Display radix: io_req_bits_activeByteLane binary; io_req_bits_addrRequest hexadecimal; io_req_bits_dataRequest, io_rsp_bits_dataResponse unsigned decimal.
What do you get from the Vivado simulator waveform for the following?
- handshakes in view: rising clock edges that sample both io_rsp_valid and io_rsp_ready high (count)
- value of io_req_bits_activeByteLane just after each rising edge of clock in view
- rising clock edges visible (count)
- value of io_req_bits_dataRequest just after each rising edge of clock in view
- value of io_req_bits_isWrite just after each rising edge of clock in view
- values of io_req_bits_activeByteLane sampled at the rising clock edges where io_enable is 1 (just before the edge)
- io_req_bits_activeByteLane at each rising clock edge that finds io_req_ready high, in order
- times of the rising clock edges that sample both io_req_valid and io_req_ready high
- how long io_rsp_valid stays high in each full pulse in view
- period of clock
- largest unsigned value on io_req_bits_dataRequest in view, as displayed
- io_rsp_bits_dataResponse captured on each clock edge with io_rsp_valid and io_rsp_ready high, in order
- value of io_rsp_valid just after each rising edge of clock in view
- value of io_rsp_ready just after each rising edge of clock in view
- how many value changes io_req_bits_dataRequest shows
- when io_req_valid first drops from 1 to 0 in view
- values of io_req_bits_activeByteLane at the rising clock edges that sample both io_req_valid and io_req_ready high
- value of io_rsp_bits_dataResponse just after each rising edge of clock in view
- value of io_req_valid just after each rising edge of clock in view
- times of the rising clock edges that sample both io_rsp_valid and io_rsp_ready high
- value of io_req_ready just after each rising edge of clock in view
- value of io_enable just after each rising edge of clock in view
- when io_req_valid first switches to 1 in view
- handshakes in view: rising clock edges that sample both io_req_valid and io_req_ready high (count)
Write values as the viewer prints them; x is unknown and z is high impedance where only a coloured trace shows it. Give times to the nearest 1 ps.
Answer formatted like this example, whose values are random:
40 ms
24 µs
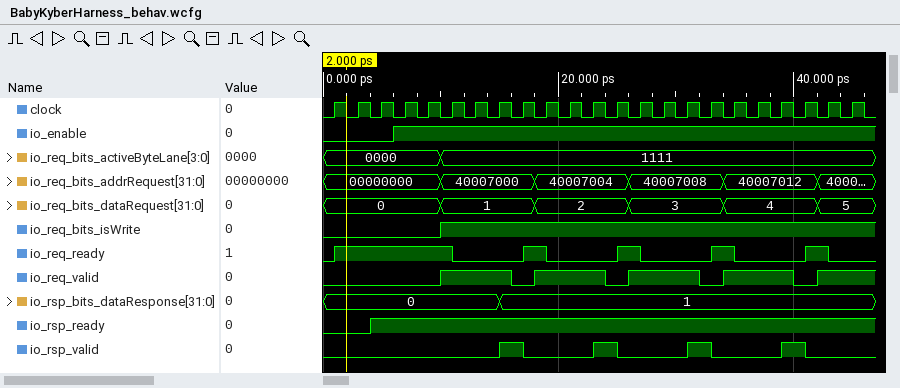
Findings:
4
0000, 0000, 0000, 0000, 0000, 1111, 1111, 1111, 1111, 1111, 1111, 1111, 1111, 1111, 1111, 1111, 1111, 1111, 1111, 1111, 1111, 1111, 1111
23
0, 0, 0, 0, 0, 1, 1, 1, 1, 2, 2, 2, 2, 3, 3, 3, 3, 4, 4, 4, 4, 5, 5
0 0 0 0 0 1 1 1 1 1 1 1 1 1 1 1 1 1 1 1 1 1 1
0000, 0000, 1111, 1111, 1111, 1111, 1111, 1111, 1111, 1111, 1111, 1111, 1111, 1111, 1111, 1111, 1111, 1111, 1111, 1111
0000, 0000, 0000, 0000, 1111, 1111, 1111, 1111, 1111
11 ps, 19 ps, 27 ps, 35 ps, 43 ps
2 ps, 2 ps, 2 ps, 2 ps
2 ps
5
1, 1, 1, 1
0 0 0 0 0 0 0 1 0 0 0 1 0 0 0 1 0 0 0 1 0 0 0
0 0 1 1 1 1 1 1 1 1 1 1 1 1 1 1 1 1 1 1 1 1 1
5
16 ps
1111, 1111, 1111, 1111, 1111
0, 0, 0, 0, 0, 0, 0, 1, 1, 1, 1, 1, 1, 1, 1, 1, 1, 1, 1, 1, 1, 1, 1
0 0 0 0 0 1 1 1 0 1 1 1 0 1 1 1 0 1 1 1 0 1 1
17 ps, 25 ps, 33 ps, 41 ps
1 1 1 1 1 0 0 0 1 0 0 0 1 0 0 0 1 0 0 0 1 0 0
0 0 0 1 1 1 1 1 1 1 1 1 1 1 1 1 1 1 1 1 1 1 1
10 ps
5
